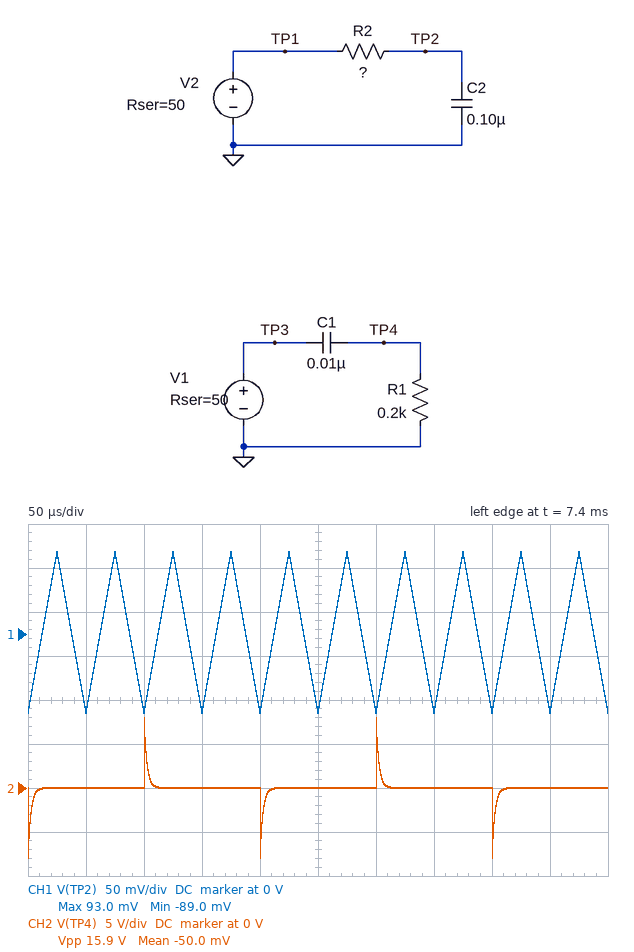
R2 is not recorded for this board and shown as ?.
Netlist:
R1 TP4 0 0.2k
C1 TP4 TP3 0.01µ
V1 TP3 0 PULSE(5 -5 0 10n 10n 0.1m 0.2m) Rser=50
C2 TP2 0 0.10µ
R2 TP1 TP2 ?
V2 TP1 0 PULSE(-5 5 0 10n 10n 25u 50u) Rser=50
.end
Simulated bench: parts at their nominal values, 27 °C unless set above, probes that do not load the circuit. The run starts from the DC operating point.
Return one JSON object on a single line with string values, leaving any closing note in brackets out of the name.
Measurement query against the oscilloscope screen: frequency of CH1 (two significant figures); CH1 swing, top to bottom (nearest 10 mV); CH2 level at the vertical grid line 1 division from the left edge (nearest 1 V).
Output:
{"frequency of CH1": "20 kHz", "CH1 swing, top to bottom": "180 mV", "CH2 level at the vertical grid line 1 division from the left edge": "0 V"}
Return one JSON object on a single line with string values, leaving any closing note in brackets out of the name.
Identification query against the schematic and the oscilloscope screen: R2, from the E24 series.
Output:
{"R2, from the E24 series": "6.8 kΩ"}
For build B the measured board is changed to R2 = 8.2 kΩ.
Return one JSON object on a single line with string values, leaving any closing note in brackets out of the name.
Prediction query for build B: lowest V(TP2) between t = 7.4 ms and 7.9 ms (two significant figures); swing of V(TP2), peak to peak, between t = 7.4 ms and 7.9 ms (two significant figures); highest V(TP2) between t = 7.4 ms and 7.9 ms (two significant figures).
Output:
{"lowest V(TP2) between t = 7.4 ms and 7.9 ms": "-74 mV", "swing of V(TP2), peak to peak, between t = 7.4 ms and 7.9 ms": "150 mV", "highest V(TP2) between t = 7.4 ms and 7.9 ms": "77 mV"}
